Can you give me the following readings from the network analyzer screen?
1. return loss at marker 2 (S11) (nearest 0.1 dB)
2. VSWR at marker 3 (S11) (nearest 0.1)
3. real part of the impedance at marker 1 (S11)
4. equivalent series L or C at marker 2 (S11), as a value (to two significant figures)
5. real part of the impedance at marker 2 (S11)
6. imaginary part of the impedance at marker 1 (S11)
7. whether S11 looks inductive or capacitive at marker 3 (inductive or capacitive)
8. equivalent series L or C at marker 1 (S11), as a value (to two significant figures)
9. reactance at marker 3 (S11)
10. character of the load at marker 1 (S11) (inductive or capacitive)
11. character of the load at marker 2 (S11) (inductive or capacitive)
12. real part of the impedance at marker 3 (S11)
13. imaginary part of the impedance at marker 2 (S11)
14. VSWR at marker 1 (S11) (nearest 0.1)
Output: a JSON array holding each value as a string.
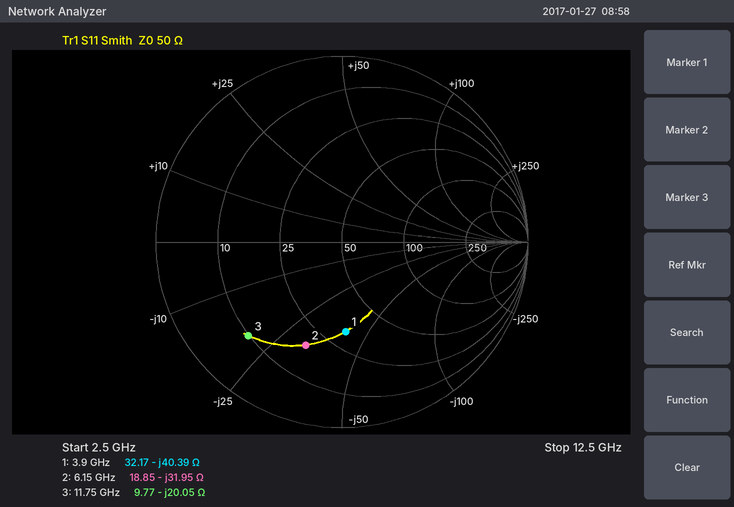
["4.6 dB", "6.0", "32.17 Ω", "810 fF", "18.85 Ω", "-40.39 Ω", "capacitive", "1.0 pF", "-20.05 Ω", "capacitive", "capacitive", "9.77 Ω", "-31.95 Ω", "2.9"]
